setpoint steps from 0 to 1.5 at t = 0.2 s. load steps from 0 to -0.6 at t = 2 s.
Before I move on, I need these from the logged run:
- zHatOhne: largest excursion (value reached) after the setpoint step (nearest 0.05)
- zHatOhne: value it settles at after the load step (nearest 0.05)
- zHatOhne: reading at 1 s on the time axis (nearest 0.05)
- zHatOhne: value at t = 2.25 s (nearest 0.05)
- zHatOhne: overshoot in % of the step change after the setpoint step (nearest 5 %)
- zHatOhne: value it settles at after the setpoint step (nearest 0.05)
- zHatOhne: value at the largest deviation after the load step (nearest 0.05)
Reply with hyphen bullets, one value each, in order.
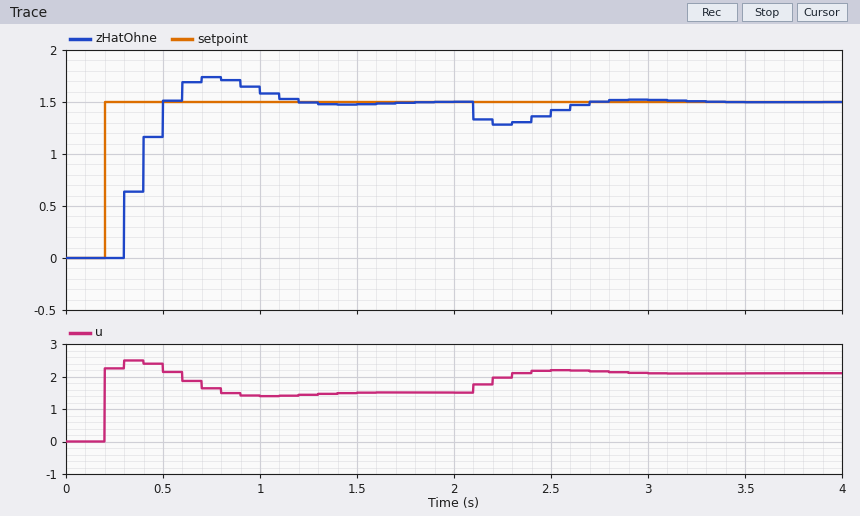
- 1.75
- 1.50
- 1.60
- 1.30
- 15 %
- 1.50
- 1.30
